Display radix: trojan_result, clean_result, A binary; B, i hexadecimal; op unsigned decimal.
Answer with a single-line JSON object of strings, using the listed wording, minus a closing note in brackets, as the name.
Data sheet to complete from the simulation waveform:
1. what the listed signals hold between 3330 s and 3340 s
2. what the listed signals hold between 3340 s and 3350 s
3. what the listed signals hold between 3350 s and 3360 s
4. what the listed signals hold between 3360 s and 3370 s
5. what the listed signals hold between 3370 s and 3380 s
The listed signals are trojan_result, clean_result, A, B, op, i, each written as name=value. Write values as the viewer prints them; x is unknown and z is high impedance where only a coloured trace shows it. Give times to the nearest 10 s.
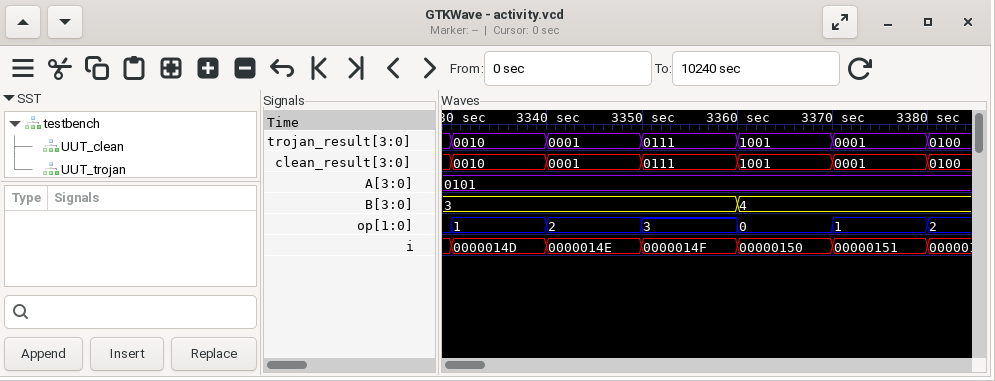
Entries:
{"what the listed signals hold between 3330 s and 3340 s": "trojan_result=0010, clean_result=0010, A=0101, B=3, op=1, i=0000014D", "what the listed signals hold between 3340 s and 3350 s": "trojan_result=0001, clean_result=0001, A=0101, B=3, op=2, i=0000014E", "what the listed signals hold between 3350 s and 3360 s": "trojan_result=0111, clean_result=0111, A=0101, B=3, op=3, i=0000014F", "what the listed signals hold between 3360 s and 3370 s": "trojan_result=1001, clean_result=1001, A=0101, B=4, op=0, i=00000150", "what the listed signals hold between 3370 s and 3380 s": "trojan_result=0001, clean_result=0001, A=0101, B=4, op=1, i=00000151"}
